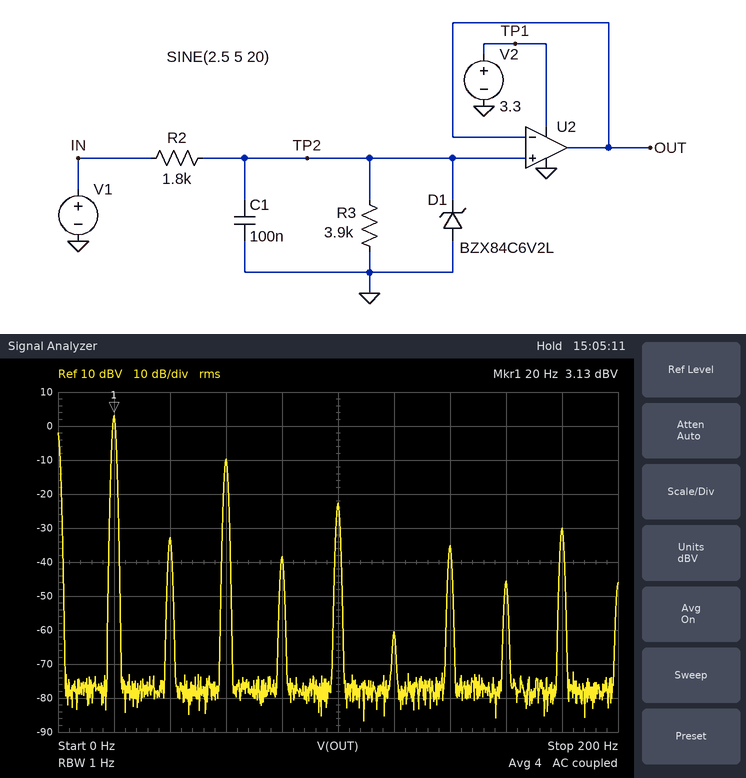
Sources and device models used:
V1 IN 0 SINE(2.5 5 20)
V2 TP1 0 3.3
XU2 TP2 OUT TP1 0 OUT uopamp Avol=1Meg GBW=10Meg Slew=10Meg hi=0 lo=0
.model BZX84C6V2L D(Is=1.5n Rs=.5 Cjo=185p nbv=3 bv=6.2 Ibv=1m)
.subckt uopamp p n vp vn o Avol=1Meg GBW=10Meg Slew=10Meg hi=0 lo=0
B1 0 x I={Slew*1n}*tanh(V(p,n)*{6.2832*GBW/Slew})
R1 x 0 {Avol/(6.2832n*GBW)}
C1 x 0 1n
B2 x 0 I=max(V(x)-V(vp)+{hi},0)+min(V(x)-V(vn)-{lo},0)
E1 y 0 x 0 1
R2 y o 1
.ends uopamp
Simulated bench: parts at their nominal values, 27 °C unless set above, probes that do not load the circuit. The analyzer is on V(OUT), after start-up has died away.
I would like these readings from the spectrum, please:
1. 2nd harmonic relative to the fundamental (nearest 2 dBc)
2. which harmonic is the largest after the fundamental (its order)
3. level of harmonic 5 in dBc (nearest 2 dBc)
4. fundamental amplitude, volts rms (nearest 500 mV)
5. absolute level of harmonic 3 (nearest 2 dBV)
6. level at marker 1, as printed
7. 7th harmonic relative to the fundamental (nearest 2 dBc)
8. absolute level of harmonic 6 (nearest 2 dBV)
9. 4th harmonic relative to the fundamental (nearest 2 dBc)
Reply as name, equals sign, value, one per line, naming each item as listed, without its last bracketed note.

2nd harmonic relative to the fundamental = -36 dBc
which harmonic is the largest after the fundamental = 3
level of harmonic 5 in dBc = -26 dBc
fundamental amplitude, volts rms = 1.5 V
absolute level of harmonic 3 = -10 dBV
level at marker 1, as printed = 3.13 dBV
7th harmonic relative to the fundamental = -38 dBc
absolute level of harmonic 6 = -60 dBV
4th harmonic relative to the fundamental = -42 dBc
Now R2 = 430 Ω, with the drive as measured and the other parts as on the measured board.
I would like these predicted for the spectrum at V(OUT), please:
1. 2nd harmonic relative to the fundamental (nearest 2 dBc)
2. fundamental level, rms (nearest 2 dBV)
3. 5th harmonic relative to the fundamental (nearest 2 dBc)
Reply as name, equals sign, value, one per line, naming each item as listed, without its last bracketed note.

2nd harmonic relative to the fundamental = -18 dBc
fundamental level, rms = 4 dBV
5th harmonic relative to the fundamental = -22 dBc
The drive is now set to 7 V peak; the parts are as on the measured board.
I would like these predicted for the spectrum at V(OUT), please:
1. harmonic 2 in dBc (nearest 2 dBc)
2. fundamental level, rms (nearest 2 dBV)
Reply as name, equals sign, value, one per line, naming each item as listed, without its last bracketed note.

harmonic 2 in dBc = -38 dBc
fundamental level, rms = 4 dBV
